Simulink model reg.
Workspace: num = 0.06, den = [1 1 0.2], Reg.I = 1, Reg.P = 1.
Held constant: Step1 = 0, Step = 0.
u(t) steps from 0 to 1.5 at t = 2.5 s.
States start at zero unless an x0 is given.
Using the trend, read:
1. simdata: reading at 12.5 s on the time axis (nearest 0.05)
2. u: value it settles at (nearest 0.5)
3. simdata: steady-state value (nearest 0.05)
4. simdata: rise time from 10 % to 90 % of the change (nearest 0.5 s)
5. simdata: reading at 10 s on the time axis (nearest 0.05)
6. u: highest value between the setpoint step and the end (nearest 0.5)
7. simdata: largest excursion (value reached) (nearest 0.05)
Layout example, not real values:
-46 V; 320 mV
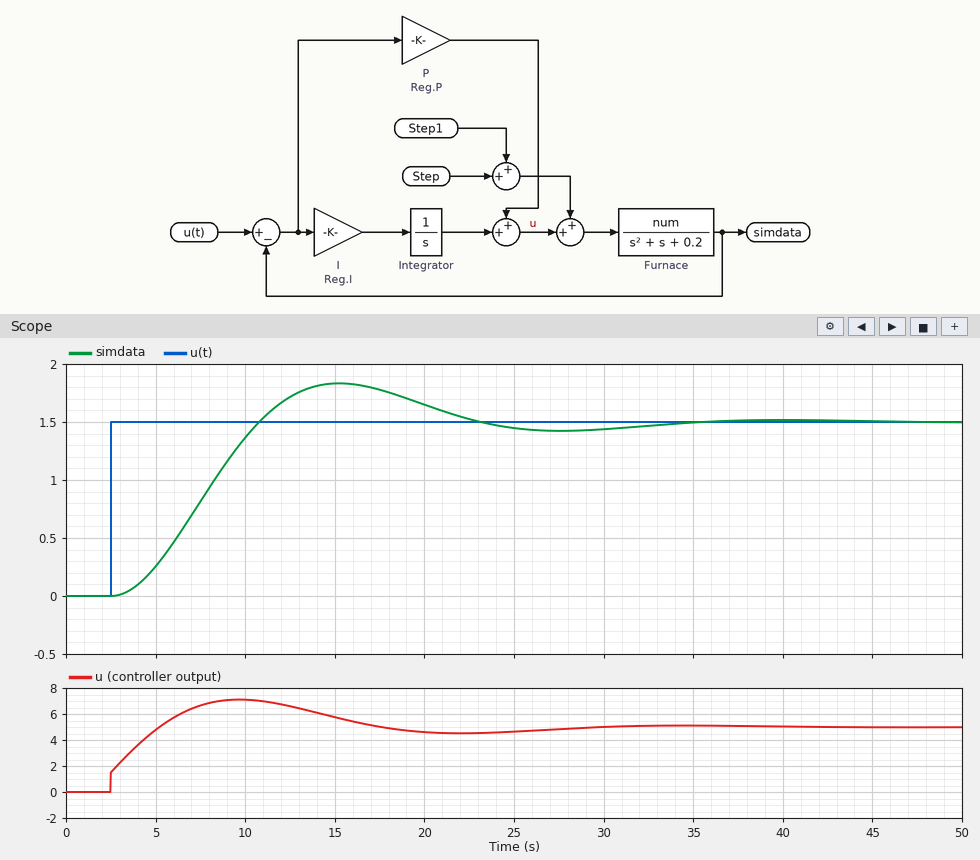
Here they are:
1.70; 5.0; 1.50; 5.5 s; 1.35; 7.0; 1.85
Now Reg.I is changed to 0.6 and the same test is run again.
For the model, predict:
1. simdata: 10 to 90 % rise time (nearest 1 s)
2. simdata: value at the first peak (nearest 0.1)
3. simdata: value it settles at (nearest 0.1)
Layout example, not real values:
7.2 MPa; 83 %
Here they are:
9 s; 1.6; 1.5
